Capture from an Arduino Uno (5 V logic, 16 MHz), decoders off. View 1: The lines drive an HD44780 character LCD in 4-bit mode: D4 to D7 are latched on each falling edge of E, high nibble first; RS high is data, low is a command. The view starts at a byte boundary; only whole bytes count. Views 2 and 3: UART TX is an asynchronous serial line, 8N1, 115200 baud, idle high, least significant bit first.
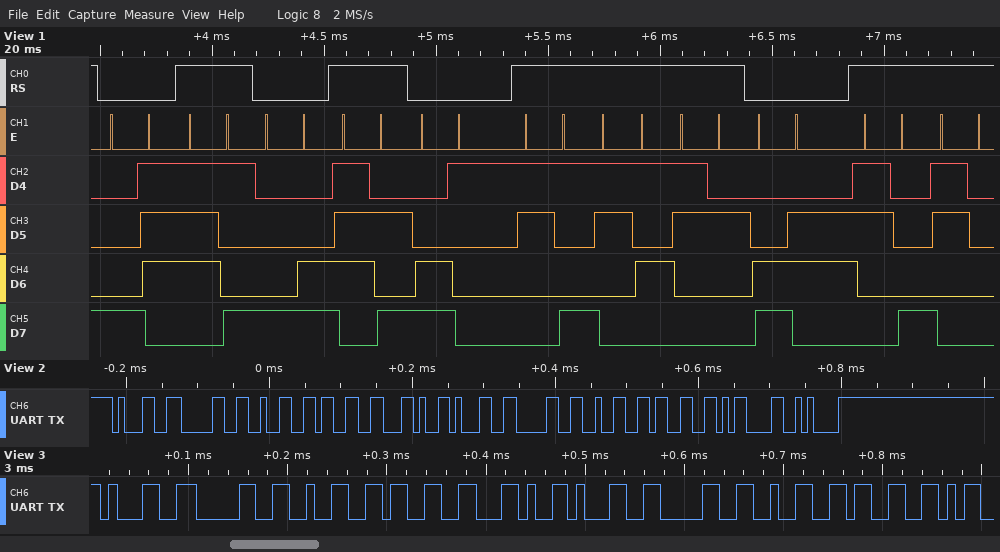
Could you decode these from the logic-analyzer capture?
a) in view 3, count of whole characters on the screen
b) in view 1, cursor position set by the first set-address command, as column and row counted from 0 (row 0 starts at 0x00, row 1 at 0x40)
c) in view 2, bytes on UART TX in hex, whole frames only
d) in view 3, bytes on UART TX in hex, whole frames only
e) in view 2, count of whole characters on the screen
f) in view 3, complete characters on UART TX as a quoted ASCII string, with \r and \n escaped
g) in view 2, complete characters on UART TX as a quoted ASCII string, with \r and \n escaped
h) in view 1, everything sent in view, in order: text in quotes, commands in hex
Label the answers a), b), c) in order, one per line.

a) 9
b) column 7, row 0
c) 31 30 32 33 2C 31 30 32 33 0D 0A
d) 31 30 32 33 2C 31 30 32 33
e) 11
f) "1023,1023"
g) "1023,1023\r\n"
h) 0x87 "y" 0x8C "z" 0xC1 "952" 0xC6 "80"
